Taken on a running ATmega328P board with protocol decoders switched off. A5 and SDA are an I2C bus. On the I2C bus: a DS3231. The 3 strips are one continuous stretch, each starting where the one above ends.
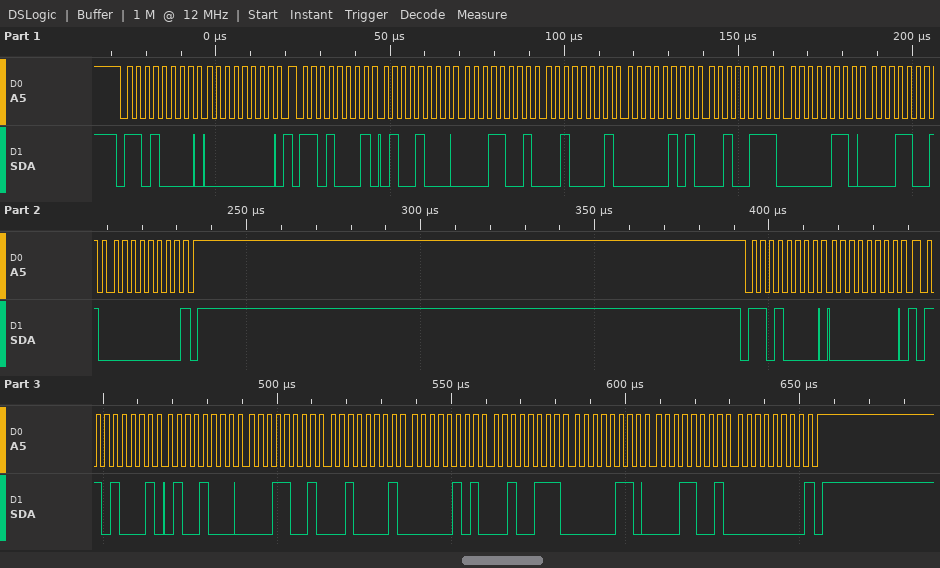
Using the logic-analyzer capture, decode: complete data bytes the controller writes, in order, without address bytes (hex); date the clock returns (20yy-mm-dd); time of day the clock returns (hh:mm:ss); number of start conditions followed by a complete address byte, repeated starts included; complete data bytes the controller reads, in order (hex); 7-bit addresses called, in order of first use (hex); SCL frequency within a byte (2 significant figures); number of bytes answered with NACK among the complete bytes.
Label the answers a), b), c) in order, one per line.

a) 00 00
b) 2019-06-27
c) 21:19:48
d) 4
e) 48 19 21 05 27 06 19 00 48 19 21 05 27 06 19 00
f) 0x68
g) 400 kHz
h) 2
